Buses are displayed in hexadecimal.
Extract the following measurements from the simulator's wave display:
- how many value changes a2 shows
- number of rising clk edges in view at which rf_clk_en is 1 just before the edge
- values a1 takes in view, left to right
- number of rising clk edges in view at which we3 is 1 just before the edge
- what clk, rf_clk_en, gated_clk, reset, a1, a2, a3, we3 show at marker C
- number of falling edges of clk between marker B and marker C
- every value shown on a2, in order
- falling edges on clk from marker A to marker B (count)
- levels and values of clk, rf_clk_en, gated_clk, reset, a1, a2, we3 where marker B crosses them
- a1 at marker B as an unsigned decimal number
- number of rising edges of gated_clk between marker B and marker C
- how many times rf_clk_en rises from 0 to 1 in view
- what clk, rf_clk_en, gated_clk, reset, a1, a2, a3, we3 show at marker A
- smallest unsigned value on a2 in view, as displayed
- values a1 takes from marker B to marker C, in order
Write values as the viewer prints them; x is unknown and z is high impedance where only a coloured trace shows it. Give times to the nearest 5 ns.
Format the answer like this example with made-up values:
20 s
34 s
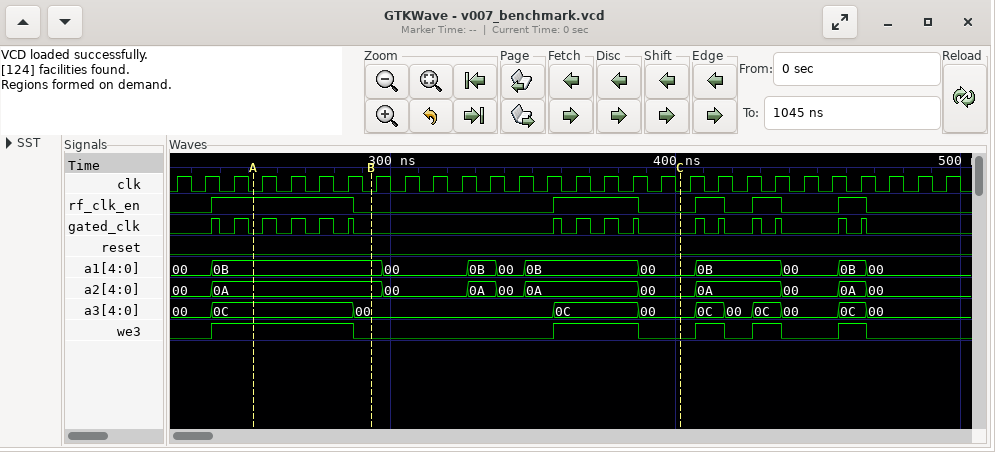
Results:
10
11
00, 0B, 00, 0B, 00, 0B, 00, 0B, 00, 0B, 00
11
clk=0, rf_clk_en=0, gated_clk=0, reset=0, a1=00, a2=00, a3=00, we3=0
11
00, 0A, 00, 0A, 00, 0A, 00, 0A, 00, 0A, 00
4
clk=0, rf_clk_en=0, gated_clk=0, reset=0, a1=0B, a2=0A, we3=0
11
4
5
clk=0, rf_clk_en=1, gated_clk=0, reset=0, a1=0B, a2=0A, a3=0C, we3=1
00
0B, 00, 0B, 00, 0B, 00
